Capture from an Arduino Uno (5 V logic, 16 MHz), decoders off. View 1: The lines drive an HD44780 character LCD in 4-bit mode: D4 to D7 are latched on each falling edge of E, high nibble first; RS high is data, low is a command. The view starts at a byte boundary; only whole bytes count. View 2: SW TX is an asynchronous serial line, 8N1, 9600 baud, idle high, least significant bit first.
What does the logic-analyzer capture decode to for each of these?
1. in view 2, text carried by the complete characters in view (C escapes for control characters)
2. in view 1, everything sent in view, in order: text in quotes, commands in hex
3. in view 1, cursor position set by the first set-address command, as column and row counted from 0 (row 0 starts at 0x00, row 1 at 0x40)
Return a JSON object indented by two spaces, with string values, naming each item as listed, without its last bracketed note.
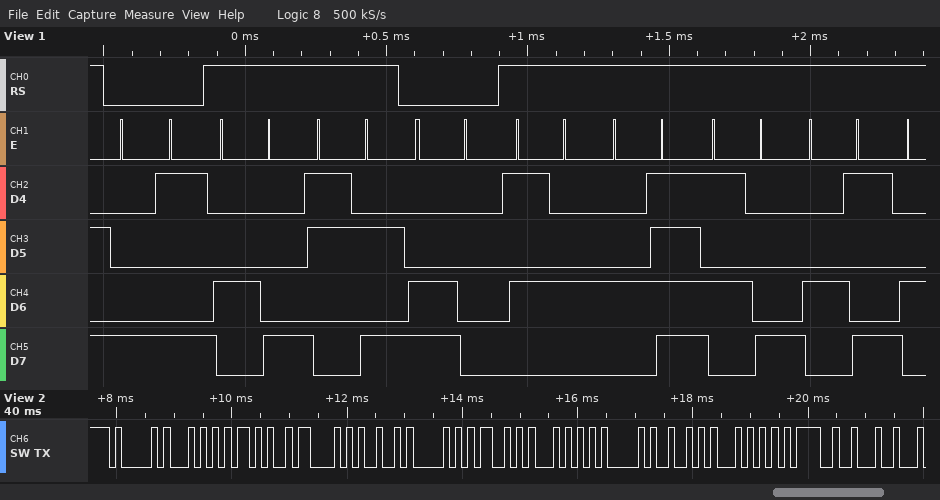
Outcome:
{
  "in view 2, text carried by the complete characters in view": "\"AT+CIPSTART=\\\"\"",
  "in view 1, everything sent in view, in order: text in quotes, commands in hex": "0x89 \"H:\" 0xC0 \"TOXI\"",
  "in view 1, cursor position set by the first set-address command, as column and row counted from 0": "column 9, row 0"
}
